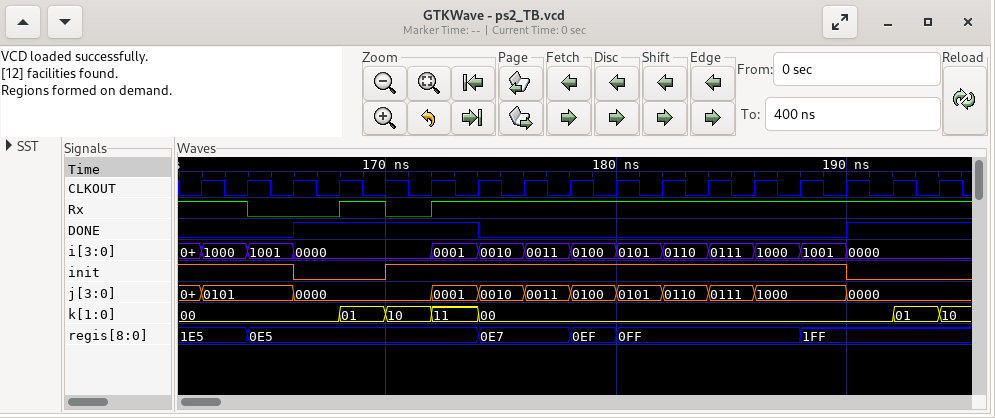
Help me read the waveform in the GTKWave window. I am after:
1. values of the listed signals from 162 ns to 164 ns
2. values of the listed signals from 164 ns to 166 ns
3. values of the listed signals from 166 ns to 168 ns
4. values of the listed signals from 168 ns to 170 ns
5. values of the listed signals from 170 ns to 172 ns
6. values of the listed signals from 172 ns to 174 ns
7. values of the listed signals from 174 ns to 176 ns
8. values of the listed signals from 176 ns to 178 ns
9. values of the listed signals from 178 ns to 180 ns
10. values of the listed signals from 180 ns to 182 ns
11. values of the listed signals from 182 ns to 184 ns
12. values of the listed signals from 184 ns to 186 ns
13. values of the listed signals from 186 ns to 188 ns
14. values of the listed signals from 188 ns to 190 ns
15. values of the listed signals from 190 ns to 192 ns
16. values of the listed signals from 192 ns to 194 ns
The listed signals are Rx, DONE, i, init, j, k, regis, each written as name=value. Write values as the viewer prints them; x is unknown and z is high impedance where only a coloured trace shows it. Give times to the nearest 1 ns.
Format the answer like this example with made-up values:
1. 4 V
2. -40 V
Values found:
1. Rx=1, DONE=0, i=1000, init=1, j=0101, k=00, regis=1E5
2. Rx=0, DONE=0, i=1001, init=1, j=0101, k=00, regis=0E5
3. Rx=0, DONE=1, i=0000, init=0, j=0000, k=00, regis=0E5
4. Rx=1, DONE=1, i=0000, init=0, j=0000, k=01, regis=0E5
5. Rx=0, DONE=1, i=0000, init=1, j=0000, k=10, regis=0E5
6. Rx=1, DONE=1, i=0001, init=1, j=0001, k=11, regis=0E5
7. Rx=1, DONE=0, i=0010, init=1, j=0010, k=00, regis=0E7
8. Rx=1, DONE=0, i=0011, init=1, j=0011, k=00, regis=0E7
9. Rx=1, DONE=0, i=0100, init=1, j=0100, k=00, regis=0EF
10. Rx=1, DONE=0, i=0101, init=1, j=0101, k=00, regis=0FF
11. Rx=1, DONE=0, i=0110, init=1, j=0110, k=00, regis=0FF
12. Rx=1, DONE=0, i=0111, init=1, j=0111, k=00, regis=0FF
13. Rx=1, DONE=0, i=1000, init=1, j=1000, k=00, regis=0FF
14. Rx=1, DONE=0, i=1001, init=1, j=1000, k=00, regis=1FF
15. Rx=1, DONE=1, i=0000, init=0, j=0000, k=00, regis=1FF
16. Rx=1, DONE=1, i=0000, init=0, j=0000, k=01, regis=1FF
